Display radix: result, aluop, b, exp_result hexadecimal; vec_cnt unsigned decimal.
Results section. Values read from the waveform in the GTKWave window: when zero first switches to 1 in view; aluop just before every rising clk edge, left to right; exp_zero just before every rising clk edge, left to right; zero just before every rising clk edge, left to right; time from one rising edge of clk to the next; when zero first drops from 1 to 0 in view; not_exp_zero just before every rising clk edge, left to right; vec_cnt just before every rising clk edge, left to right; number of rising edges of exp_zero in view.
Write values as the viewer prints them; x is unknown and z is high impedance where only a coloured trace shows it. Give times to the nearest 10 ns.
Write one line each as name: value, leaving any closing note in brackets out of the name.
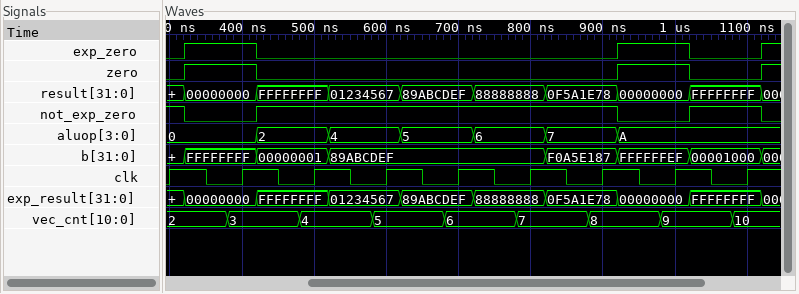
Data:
when zero first switches to 1 in view: 320 ns
aluop just before every rising clk edge, left to right: 0, 0, 2, 4, 5, 6, 7, A, A
exp_zero just before every rising clk edge, left to right: 0 1 0 0 0 0 0 1 0
zero just before every rising clk edge, left to right: 0 1 0 0 0 0 0 1 0
time from one rising edge of clk to the next: 100 ns
when zero first drops from 1 to 0 in view: 420 ns
not_exp_zero just before every rising clk edge, left to right: 1 0 1 1 1 1 1 0 1
vec_cnt just before every rising clk edge, left to right: 2, 3, 4, 5, 6, 7, 8, 9, 10
number of rising edges of exp_zero in view: 3
